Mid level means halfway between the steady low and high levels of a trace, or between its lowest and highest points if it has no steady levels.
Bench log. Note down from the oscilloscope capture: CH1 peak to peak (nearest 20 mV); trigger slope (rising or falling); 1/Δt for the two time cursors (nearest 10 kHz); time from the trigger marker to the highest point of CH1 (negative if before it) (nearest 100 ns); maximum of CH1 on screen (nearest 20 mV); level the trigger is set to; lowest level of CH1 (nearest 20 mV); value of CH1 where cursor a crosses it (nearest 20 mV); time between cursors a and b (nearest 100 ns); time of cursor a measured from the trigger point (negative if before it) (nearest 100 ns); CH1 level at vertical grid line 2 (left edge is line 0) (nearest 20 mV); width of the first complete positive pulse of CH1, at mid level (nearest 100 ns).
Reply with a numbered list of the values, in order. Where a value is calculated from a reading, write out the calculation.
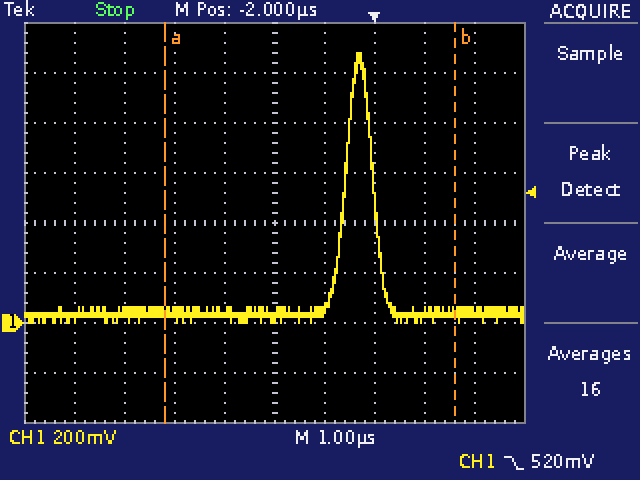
1. 1.08 V − (0 mV) = 1.08 V
2. falling
3. 1 / 5.8 µs ≈ 170 kHz
4. -300 ns
5. 1.08 V
6. 520 mV
7. 0 mV
8. 40 mV
9. 5.8 µs
10. -4.2 µs
11. 40 mV
12. 600 ns
